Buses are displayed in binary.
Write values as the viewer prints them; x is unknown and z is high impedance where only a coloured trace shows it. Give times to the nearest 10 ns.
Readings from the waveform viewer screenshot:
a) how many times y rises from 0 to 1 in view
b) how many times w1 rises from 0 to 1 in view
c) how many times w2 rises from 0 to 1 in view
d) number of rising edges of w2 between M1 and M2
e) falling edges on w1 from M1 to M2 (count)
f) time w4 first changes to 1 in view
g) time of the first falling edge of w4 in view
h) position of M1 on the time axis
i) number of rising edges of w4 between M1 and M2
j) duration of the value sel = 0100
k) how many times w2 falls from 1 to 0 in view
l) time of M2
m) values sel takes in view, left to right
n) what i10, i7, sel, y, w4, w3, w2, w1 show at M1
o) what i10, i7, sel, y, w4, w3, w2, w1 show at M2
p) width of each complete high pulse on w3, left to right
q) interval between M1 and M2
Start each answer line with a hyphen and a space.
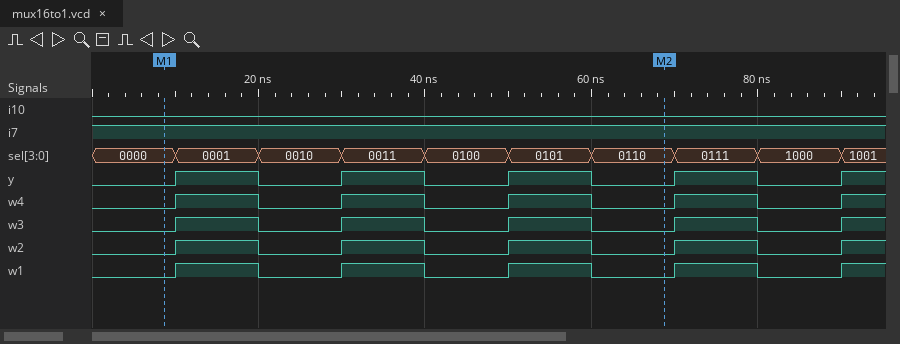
- 5
- 5
- 5
- 3
- 3
- 10 ns
- 20 ns
- 10 ns
- 3
- 10 ns
- 4
- 70 ns
- 0000, 0001, 0010, 0011, 0100, 0101, 0110, 0111, 1000, 1001
- i10=0, i7=1, sel=0000, y=0, w4=0, w3=0, w2=0, w1=0
- i10=0, i7=1, sel=0110, y=0, w4=0, w3=0, w2=0, w1=0
- 10 ns, 10 ns, 10 ns, 10 ns
- 60 ns
